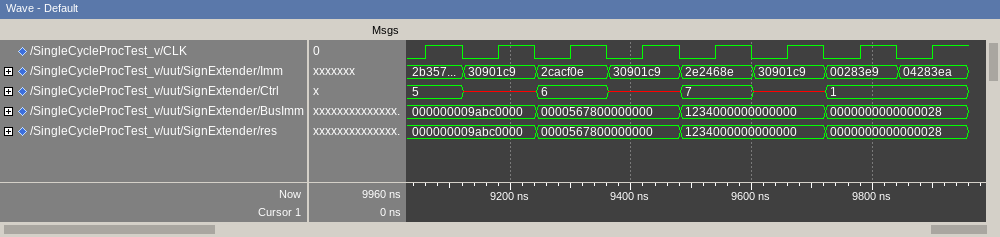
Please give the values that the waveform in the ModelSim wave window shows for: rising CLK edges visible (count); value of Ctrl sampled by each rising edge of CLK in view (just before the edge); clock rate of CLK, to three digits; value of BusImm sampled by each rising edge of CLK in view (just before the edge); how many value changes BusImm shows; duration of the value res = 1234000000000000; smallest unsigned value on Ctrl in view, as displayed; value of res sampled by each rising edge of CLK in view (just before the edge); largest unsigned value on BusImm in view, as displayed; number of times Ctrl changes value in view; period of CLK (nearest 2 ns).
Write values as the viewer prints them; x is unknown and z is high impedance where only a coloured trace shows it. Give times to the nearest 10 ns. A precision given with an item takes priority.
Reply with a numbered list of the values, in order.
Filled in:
1. 8
2. 5, x, 6, x, 7, x, 1, 1
3. 8.33 MHz
4. 000000009abc0000, 000000009abc0000, 0000567800000000, 0000567800000000, 1234000000000000, 1234000000000000, 0000000000000028, 0000000000000028
5. 3
6. 240 ns
7. 1
8. 000000009abc0000, 000000009abc0000, 0000567800000000, 0000567800000000, 1234000000000000, 1234000000000000, 0000000000000028, 0000000000000028
9. 1234000000000000
10. 6
11. 120 ns
